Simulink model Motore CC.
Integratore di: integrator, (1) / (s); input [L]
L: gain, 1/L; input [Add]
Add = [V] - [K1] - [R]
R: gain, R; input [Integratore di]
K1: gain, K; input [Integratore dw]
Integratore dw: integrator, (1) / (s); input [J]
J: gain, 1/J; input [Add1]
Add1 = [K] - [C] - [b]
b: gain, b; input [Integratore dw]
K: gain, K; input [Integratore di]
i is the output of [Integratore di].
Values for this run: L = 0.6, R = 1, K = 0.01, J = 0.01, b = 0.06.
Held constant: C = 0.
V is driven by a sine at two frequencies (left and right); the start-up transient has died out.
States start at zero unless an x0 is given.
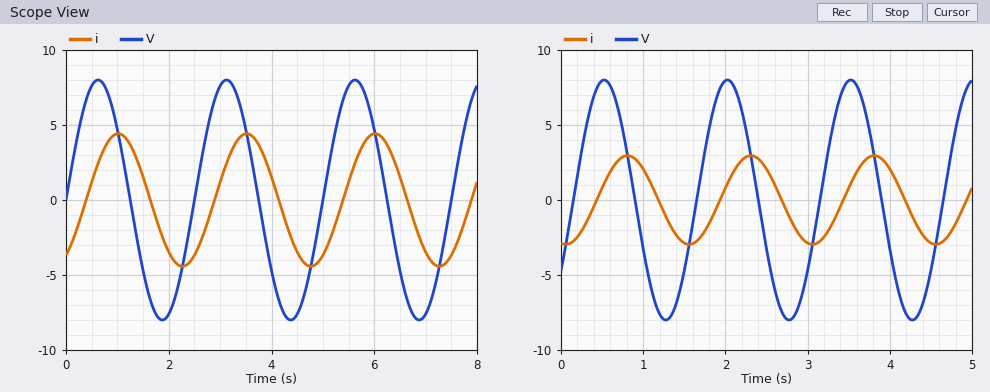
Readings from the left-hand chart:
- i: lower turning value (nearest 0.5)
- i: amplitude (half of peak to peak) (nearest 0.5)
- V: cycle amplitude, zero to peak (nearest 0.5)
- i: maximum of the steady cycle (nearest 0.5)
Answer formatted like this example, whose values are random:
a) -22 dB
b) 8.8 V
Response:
a) -4.5
b) 4.5
c) 8.0
d) 4.5
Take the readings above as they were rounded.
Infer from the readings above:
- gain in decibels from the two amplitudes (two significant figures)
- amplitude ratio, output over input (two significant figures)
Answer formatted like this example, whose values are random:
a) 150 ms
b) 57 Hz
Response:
a) -5.0 dB
b) 0.56
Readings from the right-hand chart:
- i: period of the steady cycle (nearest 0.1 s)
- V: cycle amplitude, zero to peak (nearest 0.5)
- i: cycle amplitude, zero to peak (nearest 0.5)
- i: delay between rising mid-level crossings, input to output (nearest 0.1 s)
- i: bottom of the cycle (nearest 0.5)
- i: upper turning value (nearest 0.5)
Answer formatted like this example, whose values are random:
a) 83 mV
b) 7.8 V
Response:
a) 1.5 s
b) 8.0
c) 3.0
d) 0.3 s
e) -3.0
f) 3.0
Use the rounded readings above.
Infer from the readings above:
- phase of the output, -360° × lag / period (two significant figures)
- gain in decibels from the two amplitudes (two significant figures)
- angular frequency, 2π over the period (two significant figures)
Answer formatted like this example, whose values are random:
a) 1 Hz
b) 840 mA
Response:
a) -72°
b) -8.5 dB
c) 4.2 rad/s
